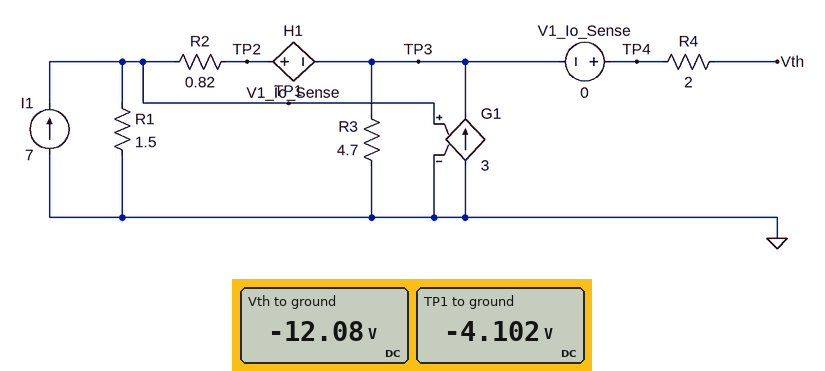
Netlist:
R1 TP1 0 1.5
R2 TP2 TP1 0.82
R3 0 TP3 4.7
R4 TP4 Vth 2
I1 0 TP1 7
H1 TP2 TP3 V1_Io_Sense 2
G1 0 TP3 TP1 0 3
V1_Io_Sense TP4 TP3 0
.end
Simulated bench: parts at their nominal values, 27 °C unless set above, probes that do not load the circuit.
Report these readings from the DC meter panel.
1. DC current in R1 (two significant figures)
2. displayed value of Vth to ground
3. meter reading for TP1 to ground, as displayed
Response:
2.7 A
-12.08 V
-4.102 V
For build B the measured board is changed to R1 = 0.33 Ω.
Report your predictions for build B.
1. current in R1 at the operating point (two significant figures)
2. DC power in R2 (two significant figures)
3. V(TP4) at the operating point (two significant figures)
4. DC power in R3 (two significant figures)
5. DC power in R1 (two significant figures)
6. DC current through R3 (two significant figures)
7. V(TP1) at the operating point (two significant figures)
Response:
32 A
520 W
31 V
210 W
340 W
6.7 A
11 V
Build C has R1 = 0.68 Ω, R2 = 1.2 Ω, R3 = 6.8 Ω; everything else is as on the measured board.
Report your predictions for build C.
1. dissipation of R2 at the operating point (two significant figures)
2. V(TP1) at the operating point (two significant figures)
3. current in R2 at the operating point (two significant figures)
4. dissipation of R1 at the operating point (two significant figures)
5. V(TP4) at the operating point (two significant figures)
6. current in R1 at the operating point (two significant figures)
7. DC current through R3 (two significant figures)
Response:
380 W
-7.3 V
18 A
79 W
-29 V
11 A
4.2 A
